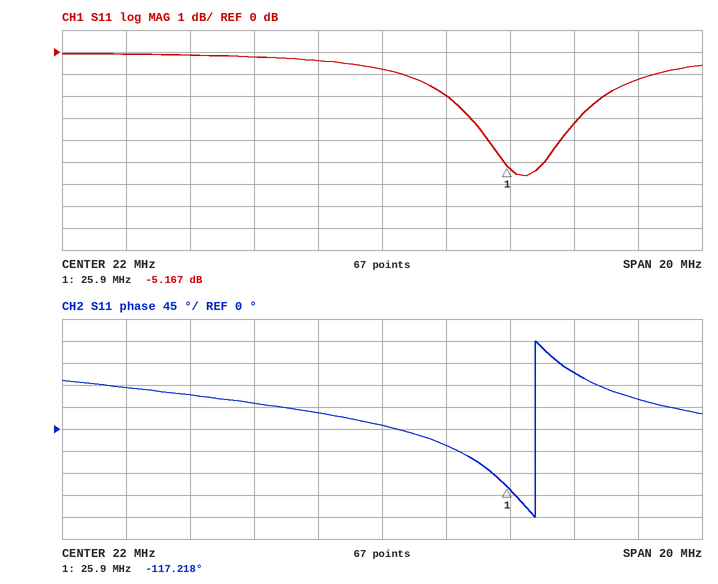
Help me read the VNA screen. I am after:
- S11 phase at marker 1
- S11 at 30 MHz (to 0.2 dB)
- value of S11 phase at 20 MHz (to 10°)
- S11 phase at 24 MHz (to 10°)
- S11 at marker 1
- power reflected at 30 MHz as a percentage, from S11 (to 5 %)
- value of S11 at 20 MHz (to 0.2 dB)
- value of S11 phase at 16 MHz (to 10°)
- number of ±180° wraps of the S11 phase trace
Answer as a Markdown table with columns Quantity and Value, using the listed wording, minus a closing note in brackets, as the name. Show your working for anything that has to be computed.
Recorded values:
| Quantity | Value |
|---|---|
| S11 phase at marker 1 | -117.218° |
| S11 at 30 MHz | -1.2 dB |
| value of S11 phase at 20 MHz | 30° |
| S11 phase at 24 MHz | -30° |
| S11 at marker 1 | -5.167 dB |
| power reflected at 30 MHz as a percentage, from S11 | 10^(-1.2/10) ≈ 75.9 %, so 75 % to the nearest 5 % |
| value of S11 at 20 MHz | -0.4 dB |
| value of S11 phase at 16 MHz | 70° |
| number of ±180° wraps of the S11 phase trace | 1 |
